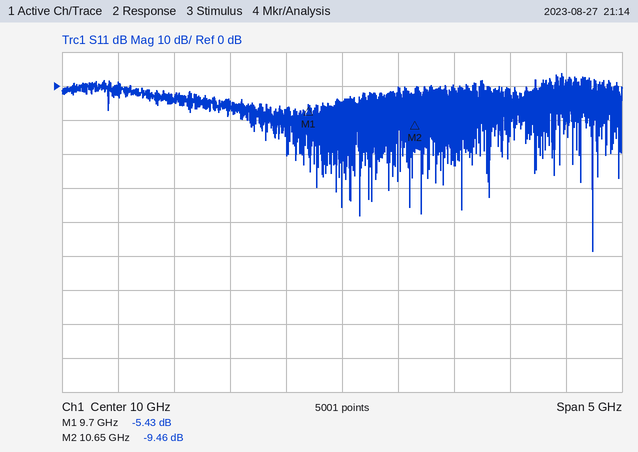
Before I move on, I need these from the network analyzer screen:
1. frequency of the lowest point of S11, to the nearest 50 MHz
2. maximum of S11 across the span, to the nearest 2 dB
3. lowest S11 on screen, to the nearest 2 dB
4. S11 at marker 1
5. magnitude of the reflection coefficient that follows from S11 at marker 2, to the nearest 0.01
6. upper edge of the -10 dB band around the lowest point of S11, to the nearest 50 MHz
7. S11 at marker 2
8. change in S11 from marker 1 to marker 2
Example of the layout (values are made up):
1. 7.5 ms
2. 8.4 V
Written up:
1. 12.25 GHz
2. 4 dB
3. -48 dB
4. -5.43 dB
5. 0.34
6. 12.25 GHz
7. -9.46 dB
8. -4.03 dB
